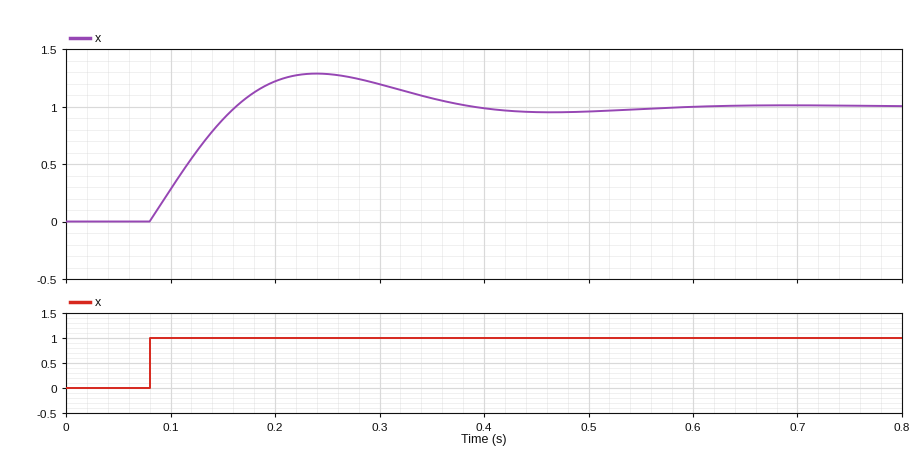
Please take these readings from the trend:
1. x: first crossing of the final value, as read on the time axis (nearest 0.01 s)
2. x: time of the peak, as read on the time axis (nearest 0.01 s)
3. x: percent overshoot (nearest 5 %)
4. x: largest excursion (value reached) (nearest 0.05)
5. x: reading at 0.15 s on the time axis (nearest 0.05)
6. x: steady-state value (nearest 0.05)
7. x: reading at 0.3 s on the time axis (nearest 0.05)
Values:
0.16 s
0.24 s
30 %
1.30
0.90
1.00
1.20
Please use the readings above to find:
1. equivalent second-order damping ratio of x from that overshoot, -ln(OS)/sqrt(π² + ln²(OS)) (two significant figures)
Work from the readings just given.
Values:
0.36
